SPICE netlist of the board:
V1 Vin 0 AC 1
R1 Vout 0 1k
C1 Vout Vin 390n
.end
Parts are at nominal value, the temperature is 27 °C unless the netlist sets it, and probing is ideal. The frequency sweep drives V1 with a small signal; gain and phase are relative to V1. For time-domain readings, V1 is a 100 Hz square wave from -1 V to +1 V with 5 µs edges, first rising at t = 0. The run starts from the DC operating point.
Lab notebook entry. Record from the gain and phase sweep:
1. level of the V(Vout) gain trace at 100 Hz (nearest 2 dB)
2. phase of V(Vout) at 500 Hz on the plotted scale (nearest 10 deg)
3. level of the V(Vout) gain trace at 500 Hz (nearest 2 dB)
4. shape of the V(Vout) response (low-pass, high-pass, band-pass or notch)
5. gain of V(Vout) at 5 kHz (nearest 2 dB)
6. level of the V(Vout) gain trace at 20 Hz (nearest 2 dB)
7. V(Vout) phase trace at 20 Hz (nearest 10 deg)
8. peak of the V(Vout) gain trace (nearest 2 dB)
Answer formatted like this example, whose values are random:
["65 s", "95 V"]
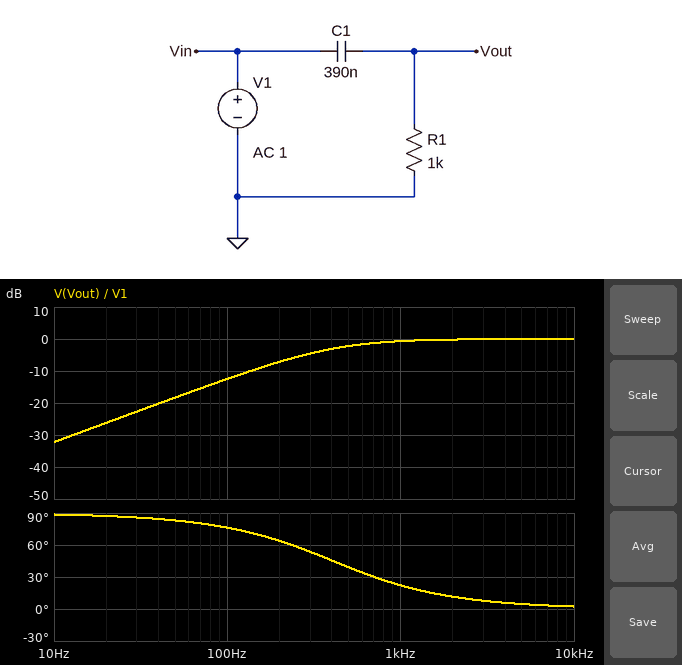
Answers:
["-12 dB", "40 deg", "-2 dB", "high-pass", "0 dB", "-26 dB", "90 deg", "0 dB"]
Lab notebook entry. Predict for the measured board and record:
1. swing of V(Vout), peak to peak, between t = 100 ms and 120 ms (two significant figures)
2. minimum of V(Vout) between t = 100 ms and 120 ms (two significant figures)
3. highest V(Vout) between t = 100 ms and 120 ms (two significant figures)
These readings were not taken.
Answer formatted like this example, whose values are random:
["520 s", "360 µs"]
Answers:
["4.0 V", "-2.0 V", "2.0 V"]
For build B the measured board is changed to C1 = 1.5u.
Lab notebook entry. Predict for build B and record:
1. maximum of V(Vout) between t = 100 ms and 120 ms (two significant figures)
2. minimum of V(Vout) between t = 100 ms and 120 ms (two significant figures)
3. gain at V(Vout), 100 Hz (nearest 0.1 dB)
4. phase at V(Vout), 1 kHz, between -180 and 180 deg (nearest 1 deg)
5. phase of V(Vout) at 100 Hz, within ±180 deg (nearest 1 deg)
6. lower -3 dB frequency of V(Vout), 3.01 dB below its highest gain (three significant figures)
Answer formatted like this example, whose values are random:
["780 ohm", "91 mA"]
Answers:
["1.9 V", "-1.9 V", "-3.3 dB", "6 deg", "47 deg", "106 Hz"]
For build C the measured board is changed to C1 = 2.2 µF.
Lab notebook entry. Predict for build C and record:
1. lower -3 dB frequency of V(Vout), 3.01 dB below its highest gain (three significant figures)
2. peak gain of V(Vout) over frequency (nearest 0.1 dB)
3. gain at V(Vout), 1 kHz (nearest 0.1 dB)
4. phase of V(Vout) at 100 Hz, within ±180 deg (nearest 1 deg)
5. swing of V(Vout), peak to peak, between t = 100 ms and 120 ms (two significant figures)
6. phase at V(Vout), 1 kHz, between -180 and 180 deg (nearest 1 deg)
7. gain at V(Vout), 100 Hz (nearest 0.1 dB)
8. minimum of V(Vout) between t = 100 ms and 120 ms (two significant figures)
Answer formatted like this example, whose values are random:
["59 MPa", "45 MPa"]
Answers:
["72.3 Hz", "0 dB", "0 dB", "36 deg", "3.6 V", "4 deg", "-1.8 dB", "-1.8 V"]
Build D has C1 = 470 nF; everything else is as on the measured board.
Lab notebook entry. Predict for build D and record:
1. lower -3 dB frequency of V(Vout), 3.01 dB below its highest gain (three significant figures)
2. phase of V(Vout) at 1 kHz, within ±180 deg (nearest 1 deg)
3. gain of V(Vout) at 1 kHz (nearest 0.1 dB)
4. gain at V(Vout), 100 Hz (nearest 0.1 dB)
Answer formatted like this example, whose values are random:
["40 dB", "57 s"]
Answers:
["339 Hz", "19 deg", "-0.5 dB", "-11.0 dB"]
